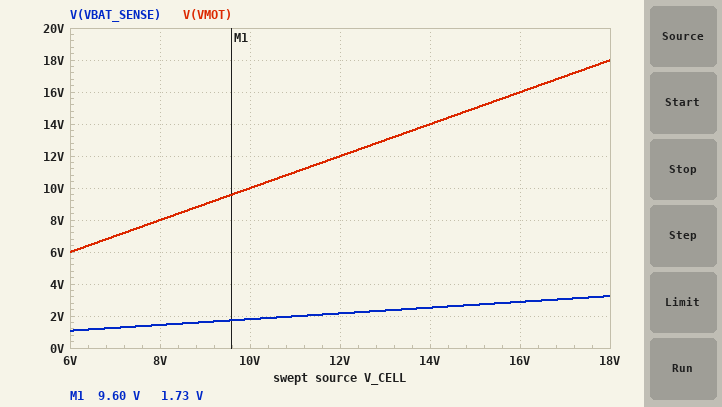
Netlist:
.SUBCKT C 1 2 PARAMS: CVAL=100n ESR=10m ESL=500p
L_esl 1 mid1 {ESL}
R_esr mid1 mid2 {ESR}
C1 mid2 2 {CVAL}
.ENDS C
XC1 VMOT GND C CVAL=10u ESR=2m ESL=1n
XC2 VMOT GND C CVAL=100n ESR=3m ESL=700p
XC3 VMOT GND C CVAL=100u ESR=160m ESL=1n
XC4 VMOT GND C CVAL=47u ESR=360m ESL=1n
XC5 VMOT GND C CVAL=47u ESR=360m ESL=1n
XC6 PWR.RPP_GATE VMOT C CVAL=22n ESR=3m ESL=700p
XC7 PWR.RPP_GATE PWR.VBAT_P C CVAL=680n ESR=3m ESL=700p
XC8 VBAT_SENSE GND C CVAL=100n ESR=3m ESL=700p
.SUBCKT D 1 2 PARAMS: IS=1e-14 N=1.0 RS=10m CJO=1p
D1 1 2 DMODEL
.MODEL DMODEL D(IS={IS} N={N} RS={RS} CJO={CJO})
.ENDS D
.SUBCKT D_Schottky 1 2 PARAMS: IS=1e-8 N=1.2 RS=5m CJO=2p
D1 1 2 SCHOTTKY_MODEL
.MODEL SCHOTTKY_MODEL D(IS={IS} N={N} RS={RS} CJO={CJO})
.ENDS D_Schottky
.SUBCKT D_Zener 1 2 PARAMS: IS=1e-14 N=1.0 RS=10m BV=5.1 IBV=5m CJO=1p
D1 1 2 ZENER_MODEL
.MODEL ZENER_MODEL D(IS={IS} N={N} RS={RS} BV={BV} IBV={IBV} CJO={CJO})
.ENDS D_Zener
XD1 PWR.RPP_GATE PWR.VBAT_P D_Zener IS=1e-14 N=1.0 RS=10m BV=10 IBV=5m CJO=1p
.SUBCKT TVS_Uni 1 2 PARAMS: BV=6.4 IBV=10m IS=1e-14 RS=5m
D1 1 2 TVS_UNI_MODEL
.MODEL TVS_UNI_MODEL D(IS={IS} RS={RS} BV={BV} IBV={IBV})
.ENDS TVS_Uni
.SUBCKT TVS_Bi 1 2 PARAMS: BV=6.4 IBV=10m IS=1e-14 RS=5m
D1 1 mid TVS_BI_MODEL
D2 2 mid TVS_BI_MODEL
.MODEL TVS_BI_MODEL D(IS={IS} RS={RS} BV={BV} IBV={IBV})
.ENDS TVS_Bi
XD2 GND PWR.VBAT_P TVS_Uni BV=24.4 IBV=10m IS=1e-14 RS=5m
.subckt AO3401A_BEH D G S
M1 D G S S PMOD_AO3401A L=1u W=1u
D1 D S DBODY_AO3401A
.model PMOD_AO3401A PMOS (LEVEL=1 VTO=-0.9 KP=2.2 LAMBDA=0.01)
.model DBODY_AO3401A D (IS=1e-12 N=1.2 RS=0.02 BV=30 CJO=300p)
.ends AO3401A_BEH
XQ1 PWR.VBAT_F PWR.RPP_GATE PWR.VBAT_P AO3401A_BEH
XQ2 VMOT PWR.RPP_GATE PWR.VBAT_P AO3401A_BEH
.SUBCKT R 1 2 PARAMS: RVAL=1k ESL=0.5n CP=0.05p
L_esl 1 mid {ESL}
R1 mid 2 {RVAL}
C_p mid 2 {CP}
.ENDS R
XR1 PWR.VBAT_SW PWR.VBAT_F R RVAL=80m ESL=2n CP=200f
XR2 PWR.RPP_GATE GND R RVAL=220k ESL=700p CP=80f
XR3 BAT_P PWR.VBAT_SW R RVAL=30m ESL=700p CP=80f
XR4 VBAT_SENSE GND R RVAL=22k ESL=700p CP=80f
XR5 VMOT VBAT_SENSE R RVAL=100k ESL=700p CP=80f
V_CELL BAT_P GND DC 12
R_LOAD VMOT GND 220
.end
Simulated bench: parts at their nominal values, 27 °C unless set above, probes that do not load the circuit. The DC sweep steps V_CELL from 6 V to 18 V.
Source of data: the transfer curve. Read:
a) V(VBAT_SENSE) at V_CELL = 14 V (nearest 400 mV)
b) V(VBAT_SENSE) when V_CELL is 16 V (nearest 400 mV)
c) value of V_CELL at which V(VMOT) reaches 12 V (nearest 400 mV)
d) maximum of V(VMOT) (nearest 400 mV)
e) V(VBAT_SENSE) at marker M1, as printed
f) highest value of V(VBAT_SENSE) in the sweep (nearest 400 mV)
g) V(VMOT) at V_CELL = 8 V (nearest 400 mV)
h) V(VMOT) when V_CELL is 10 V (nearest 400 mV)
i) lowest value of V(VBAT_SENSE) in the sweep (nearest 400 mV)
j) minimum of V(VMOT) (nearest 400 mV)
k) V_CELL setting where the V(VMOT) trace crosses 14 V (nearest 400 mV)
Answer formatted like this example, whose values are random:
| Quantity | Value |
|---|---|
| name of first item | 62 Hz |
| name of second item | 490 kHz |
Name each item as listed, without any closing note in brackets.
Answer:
| Quantity | Value |
|---|---|
| V(VBAT_SENSE) at V_CELL = 14 V | 2.4 V |
| V(VBAT_SENSE) when V_CELL is 16 V | 2.8 V |
| value of V_CELL at which V(VMOT) reaches 12 V | 12.0 V |
| maximum of V(VMOT) | 18.0 V |
| V(VBAT_SENSE) at marker M1, as printed | 1.73 V |
| highest value of V(VBAT_SENSE) in the sweep | 3.2 V |
| V(VMOT) at V_CELL = 8 V | 8.0 V |
| V(VMOT) when V_CELL is 10 V | 10.0 V |
| lowest value of V(VBAT_SENSE) in the sweep | 1.2 V |
| minimum of V(VMOT) | 6.0 V |
| V_CELL setting where the V(VMOT) trace crosses 14 V | 14.0 V |
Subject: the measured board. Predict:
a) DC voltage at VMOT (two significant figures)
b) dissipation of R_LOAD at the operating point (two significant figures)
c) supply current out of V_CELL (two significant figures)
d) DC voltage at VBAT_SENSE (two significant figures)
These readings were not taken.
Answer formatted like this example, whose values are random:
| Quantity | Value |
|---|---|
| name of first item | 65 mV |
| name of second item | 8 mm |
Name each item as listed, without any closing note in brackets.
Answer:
| Quantity | Value |
|---|---|
| DC voltage at VMOT | 12 V |
| dissipation of R_LOAD at the operating point | 650 mW |
| supply current out of V_CELL | 55 mA |
| DC voltage at VBAT_SENSE | 2.2 V |
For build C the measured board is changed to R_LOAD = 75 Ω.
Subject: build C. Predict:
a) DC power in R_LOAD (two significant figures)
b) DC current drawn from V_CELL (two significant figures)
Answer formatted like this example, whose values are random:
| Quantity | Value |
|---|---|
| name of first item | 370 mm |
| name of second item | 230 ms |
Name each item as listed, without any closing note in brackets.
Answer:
| Quantity | Value |
|---|---|
| DC power in R_LOAD | 1.9 W |
| DC current drawn from V_CELL | 160 mA |
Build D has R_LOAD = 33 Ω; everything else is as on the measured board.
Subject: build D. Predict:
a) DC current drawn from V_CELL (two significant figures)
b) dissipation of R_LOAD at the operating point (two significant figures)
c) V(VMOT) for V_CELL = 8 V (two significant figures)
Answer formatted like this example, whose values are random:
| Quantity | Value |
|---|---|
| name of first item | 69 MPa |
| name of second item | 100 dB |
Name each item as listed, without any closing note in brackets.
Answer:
| Quantity | Value |
|---|---|
| DC current drawn from V_CELL | 360 mA |
| dissipation of R_LOAD at the operating point | 4.3 W |
| V(VMOT) for V_CELL = 8 V | 7.9 V |
